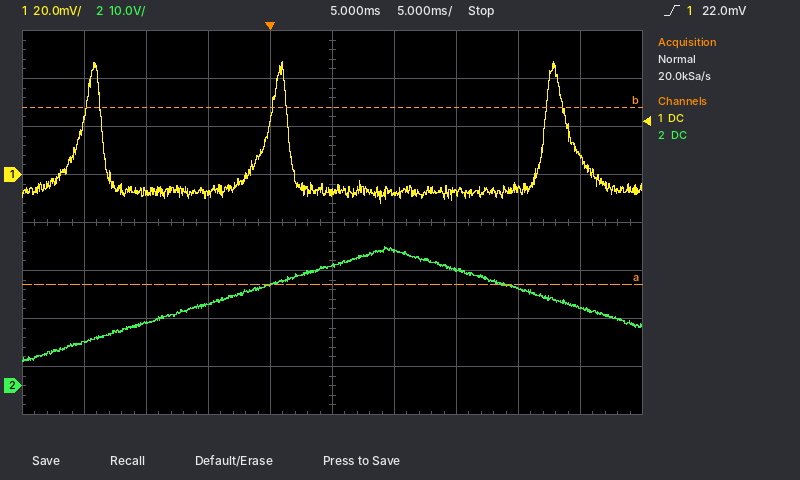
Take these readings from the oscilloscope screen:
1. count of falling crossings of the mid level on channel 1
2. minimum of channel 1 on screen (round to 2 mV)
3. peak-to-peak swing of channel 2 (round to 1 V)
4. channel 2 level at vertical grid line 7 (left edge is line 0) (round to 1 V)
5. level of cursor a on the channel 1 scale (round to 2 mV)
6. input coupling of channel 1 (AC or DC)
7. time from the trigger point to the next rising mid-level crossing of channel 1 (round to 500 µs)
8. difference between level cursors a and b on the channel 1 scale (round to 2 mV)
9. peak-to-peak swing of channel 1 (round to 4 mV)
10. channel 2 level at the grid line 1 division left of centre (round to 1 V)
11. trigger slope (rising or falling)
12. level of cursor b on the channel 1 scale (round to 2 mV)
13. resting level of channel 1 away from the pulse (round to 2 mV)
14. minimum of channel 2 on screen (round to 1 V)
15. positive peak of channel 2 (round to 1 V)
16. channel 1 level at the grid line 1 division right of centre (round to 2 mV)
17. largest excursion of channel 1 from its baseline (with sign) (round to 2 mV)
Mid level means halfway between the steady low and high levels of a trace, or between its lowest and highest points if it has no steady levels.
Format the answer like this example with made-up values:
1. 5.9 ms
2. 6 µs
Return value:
1. 3
2. -12 mV
3. 24 V
4. 24 V
5. -46 mV
6. DC
7. 22.0 ms
8. 74 mV
9. 60 mV
10. 21 V
11. rising
12. 28 mV
13. -6 mV
14. 5 V
15. 29 V
16. -8 mV
17. +54 mV
